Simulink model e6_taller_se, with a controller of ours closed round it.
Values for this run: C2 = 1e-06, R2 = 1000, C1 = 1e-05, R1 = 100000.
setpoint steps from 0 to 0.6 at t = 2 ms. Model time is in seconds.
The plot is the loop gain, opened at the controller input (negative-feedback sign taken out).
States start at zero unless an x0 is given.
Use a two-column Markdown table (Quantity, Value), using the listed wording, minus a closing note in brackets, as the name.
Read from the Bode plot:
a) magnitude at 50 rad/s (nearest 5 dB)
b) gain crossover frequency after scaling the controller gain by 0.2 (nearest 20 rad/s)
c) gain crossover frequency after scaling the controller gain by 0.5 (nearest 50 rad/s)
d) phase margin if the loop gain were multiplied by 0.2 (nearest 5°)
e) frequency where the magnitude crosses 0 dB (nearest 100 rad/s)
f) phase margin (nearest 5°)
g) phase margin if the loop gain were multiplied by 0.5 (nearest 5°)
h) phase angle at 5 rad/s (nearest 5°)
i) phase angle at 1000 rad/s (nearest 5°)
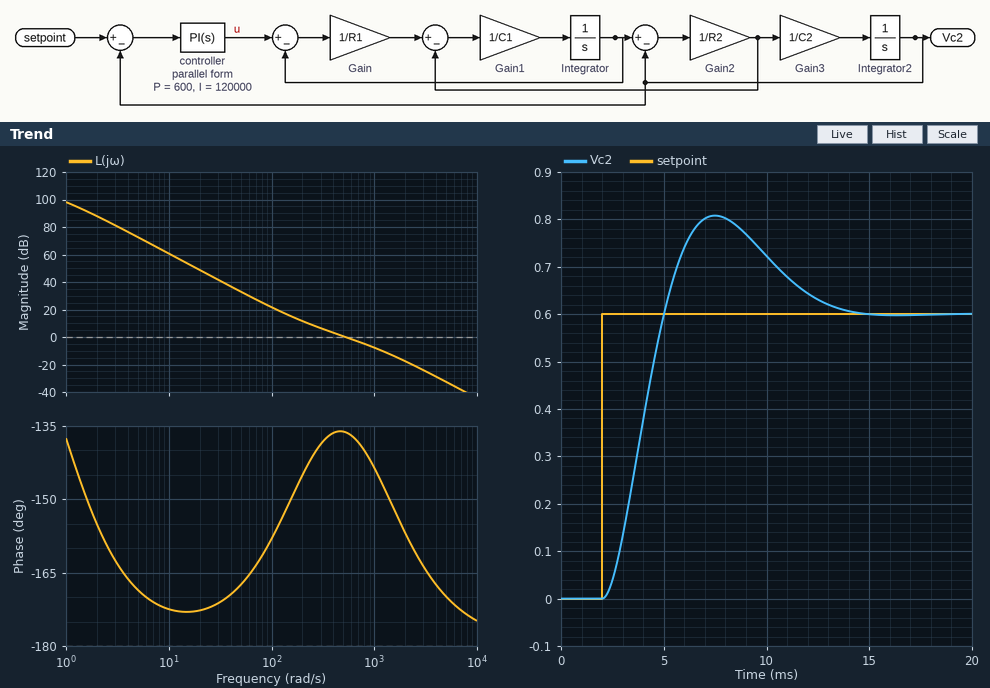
| Quantity | Value |
|---|---|
| magnitude at 50 rad/s | 35 dB |
| gain crossover frequency after scaling the controller gain by 0.2 | 160 rad/s |
| gain crossover frequency after scaling the controller gain by 0.5 | 300 rad/s |
| phase margin if the loop gain were multiplied by 0.2 | 30° |
| frequency where the magnitude crosses 0 dB | 500 rad/s |
| phase margin | 45° |
| phase margin if the loop gain were multiplied by 0.5 | 40° |
| phase angle at 5 rad/s | -170° |
| phase angle at 1000 rad/s | -145° |
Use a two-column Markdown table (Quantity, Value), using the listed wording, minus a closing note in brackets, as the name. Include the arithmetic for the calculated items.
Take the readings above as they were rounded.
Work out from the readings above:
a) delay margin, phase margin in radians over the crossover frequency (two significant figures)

| Quantity | Value |
|---|---|
| delay margin, phase margin in radians over the crossover frequency | 45 × π / 180 / 500 = 0.0016 s |
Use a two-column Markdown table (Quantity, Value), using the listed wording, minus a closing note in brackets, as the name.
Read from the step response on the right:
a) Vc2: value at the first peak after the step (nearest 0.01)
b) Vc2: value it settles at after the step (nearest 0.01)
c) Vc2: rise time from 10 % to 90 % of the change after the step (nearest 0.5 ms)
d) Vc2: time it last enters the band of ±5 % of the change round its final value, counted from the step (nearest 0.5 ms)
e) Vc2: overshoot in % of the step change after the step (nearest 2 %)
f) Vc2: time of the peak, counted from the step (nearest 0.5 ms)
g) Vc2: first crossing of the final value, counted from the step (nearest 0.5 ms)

| Quantity | Value |
|---|---|
| Vc2: value at the first peak after the step | 0.81 |
| Vc2: value it settles at after the step | 0.60 |
| Vc2: rise time from 10 % to 90 % of the change after the step | 2.0 ms |
| Vc2: time it last enters the band of ±5 % of the change round its final value, counted from the step | 10.5 ms |
| Vc2: overshoot in % of the step change after the step | 34 % |
| Vc2: time of the peak, counted from the step | 5.5 ms |
| Vc2: first crossing of the final value, counted from the step | 3.0 ms |
